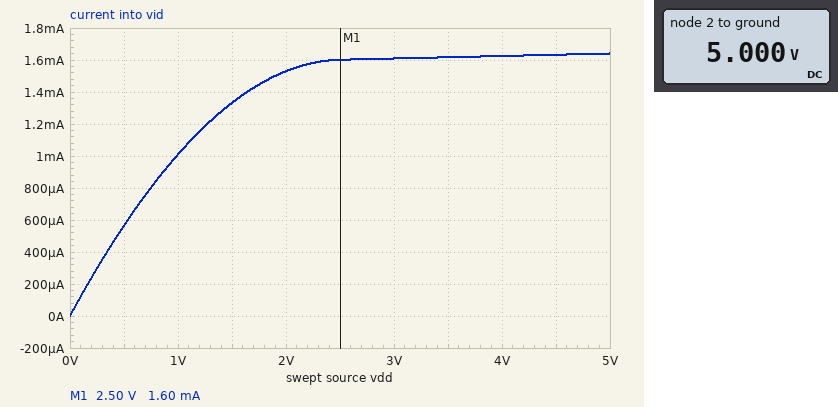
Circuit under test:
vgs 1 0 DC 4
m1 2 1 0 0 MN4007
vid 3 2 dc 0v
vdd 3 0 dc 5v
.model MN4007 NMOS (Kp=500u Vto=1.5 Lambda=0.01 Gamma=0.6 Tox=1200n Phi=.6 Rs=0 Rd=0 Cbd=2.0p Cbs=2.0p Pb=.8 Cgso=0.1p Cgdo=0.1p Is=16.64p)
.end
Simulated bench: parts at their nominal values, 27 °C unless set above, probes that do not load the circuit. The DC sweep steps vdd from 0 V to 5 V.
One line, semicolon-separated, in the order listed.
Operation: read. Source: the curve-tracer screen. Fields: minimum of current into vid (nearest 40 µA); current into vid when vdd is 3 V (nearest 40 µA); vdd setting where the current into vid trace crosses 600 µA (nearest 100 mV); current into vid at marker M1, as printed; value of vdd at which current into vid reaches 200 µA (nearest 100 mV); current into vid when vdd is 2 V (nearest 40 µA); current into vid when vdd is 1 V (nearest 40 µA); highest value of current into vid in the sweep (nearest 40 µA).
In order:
0 A; 1.60 mA; 500 mV; 1.60 mA; 200 mV; 1.52 mA; 1.00 mA; 1.64 mA
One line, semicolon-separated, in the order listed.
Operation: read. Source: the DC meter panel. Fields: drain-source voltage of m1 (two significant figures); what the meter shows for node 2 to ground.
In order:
5.0 V; 5.000 V
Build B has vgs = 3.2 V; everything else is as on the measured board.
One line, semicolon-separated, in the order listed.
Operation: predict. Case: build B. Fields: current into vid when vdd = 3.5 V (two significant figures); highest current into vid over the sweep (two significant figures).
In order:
750 µA; 760 µA
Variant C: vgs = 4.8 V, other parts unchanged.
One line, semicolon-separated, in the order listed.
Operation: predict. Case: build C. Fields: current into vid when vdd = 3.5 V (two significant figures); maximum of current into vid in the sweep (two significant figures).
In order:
2.8 mA; 2.9 mA
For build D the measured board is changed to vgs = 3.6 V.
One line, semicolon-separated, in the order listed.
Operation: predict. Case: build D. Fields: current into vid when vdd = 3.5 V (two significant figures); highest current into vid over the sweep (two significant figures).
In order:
1.1 mA; 1.2 mA
